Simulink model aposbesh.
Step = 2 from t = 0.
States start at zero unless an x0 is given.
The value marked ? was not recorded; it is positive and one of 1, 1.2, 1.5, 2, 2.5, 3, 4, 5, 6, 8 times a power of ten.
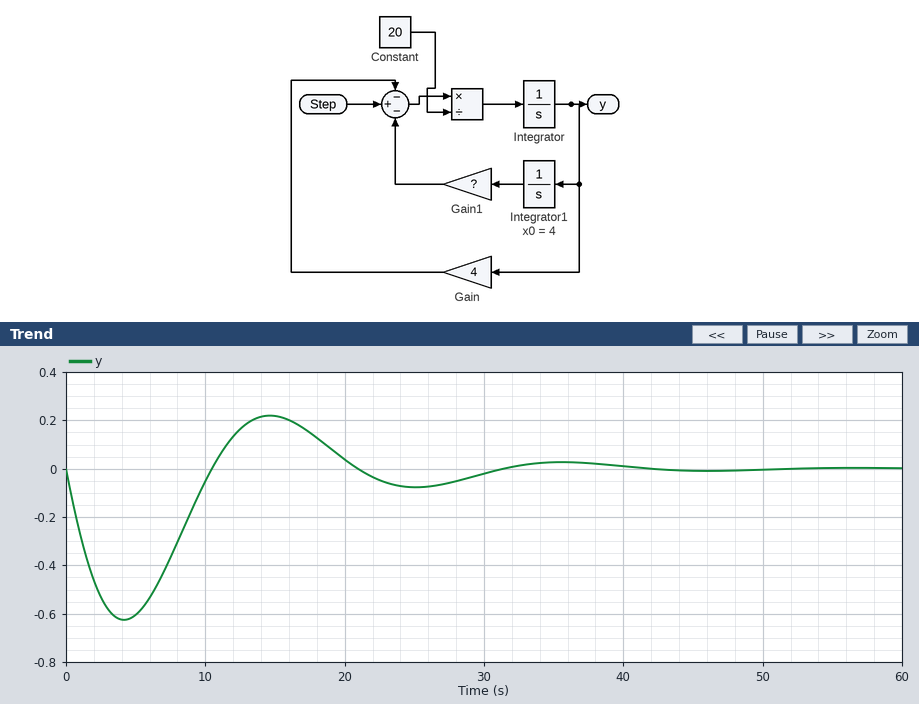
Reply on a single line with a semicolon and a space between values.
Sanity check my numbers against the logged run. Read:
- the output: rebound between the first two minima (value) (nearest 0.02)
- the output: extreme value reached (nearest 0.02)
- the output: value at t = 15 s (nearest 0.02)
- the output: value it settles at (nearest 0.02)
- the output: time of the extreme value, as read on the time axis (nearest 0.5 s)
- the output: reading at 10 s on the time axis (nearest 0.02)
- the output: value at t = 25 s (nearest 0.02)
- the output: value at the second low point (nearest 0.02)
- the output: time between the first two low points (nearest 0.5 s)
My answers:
0.22; -0.62; 0.22; 0.00; 4.0 s; -0.06; -0.08; -0.08; 21.0 s
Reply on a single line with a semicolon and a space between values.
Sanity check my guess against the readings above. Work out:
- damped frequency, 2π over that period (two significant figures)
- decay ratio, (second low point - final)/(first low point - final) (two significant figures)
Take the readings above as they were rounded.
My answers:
0.30 rad/s; 0.13
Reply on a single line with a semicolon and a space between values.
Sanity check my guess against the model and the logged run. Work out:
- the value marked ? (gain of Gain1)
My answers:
2
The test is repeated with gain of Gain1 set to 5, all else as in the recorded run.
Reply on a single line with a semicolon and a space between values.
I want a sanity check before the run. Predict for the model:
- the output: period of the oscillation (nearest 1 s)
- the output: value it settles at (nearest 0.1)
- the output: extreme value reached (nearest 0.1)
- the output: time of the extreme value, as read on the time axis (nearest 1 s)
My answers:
13 s; 0.0; -1.4; 3 s
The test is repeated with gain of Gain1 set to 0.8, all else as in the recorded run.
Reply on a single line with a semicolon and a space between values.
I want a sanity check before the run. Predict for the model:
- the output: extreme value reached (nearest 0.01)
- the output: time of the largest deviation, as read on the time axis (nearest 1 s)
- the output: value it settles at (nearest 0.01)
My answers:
-0.16; 6 s; 0.00
